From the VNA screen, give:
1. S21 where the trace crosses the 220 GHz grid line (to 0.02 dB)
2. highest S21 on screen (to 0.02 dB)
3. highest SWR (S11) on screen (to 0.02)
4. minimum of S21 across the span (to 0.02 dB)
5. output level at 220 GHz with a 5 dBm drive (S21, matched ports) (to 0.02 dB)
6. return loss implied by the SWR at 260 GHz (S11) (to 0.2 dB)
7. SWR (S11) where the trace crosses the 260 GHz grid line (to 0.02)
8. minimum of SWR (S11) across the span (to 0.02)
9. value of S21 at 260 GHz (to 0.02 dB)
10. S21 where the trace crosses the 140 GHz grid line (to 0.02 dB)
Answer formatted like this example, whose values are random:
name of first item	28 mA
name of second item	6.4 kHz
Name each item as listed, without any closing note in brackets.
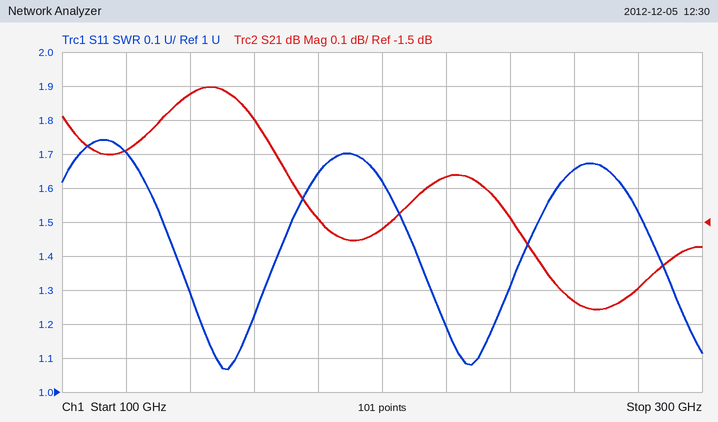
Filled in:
S21 where the trace crosses the 220 GHz grid line	-1.36 dB
highest S21 on screen	-1.10 dB
highest SWR (S11) on screen	1.74
minimum of S21 across the span	-1.76 dB
output level at 220 GHz with a 5 dBm drive (S21, matched ports)	3.64 dBm
return loss implied by the SWR at 260 GHz (S11)	12.2 dB
SWR (S11) where the trace crosses the 260 GHz grid line	1.66
minimum of SWR (S11) across the span	1.06
value of S21 at 260 GHz	-1.74 dB
S21 where the trace crosses the 140 GHz grid line	-1.12 dB
